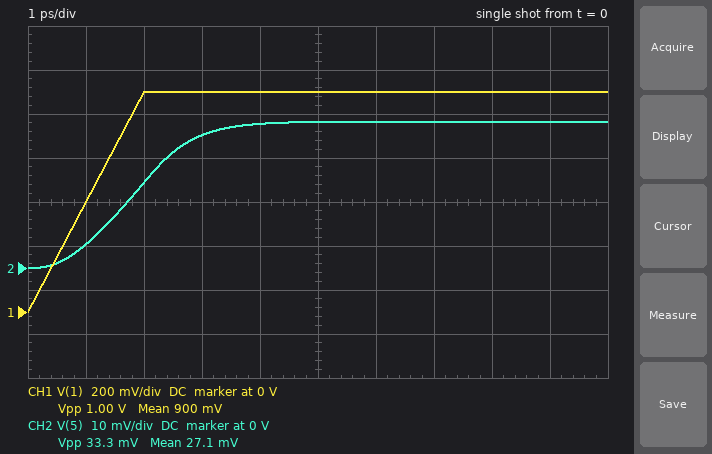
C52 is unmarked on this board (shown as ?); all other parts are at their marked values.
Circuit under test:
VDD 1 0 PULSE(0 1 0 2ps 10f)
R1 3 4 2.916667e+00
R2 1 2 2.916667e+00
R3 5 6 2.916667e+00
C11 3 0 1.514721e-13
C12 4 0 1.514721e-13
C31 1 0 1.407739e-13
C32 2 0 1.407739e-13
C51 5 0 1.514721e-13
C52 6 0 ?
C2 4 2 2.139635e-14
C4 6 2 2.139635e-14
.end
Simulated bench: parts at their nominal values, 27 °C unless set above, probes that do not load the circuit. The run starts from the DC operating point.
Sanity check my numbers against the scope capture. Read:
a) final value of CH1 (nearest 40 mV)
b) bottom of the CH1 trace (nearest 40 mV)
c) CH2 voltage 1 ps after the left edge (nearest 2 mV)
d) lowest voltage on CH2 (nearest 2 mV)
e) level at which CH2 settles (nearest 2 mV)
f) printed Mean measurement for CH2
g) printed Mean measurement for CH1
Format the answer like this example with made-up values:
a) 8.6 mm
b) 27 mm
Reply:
a) 1.00 V
b) 0 V
c) 6 mV
d) 0 V
e) 34 mV
f) 27.1 mV
g) 900 mV
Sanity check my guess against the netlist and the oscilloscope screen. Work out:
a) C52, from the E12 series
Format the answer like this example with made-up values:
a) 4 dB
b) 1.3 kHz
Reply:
a) 470 fF
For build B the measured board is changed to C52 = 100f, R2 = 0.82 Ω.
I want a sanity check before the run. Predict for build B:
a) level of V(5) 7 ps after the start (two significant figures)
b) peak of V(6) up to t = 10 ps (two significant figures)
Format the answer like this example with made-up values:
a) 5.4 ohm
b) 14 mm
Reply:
a) 78 mV
b) 84 mV
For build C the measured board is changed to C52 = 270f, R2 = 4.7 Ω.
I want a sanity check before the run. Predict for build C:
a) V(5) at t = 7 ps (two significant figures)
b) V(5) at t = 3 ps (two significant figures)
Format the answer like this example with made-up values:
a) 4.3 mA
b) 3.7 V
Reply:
a) 48 mV
b) 40 mV
